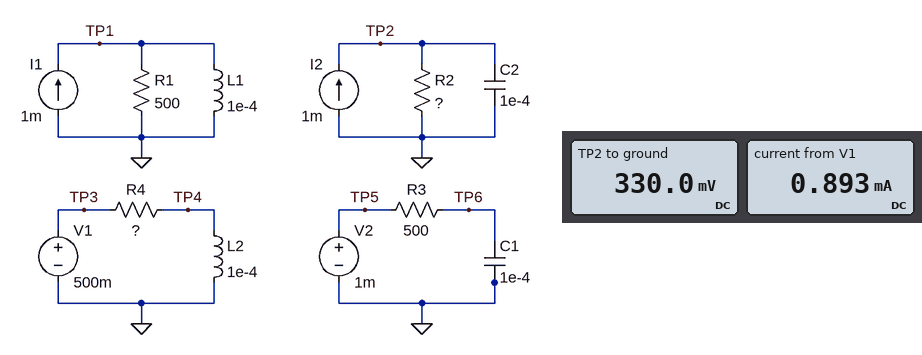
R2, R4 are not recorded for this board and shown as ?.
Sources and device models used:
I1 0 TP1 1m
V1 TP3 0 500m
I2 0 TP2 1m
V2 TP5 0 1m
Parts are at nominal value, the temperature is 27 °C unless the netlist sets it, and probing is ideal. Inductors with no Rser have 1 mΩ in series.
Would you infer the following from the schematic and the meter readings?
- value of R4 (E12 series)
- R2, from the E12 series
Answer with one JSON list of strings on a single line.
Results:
["560 Ω", "330 Ω"]
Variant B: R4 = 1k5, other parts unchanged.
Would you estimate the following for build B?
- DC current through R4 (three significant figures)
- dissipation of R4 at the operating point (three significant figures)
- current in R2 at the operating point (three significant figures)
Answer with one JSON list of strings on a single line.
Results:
["333 µA", "167 µW", "1.00 mA"]
